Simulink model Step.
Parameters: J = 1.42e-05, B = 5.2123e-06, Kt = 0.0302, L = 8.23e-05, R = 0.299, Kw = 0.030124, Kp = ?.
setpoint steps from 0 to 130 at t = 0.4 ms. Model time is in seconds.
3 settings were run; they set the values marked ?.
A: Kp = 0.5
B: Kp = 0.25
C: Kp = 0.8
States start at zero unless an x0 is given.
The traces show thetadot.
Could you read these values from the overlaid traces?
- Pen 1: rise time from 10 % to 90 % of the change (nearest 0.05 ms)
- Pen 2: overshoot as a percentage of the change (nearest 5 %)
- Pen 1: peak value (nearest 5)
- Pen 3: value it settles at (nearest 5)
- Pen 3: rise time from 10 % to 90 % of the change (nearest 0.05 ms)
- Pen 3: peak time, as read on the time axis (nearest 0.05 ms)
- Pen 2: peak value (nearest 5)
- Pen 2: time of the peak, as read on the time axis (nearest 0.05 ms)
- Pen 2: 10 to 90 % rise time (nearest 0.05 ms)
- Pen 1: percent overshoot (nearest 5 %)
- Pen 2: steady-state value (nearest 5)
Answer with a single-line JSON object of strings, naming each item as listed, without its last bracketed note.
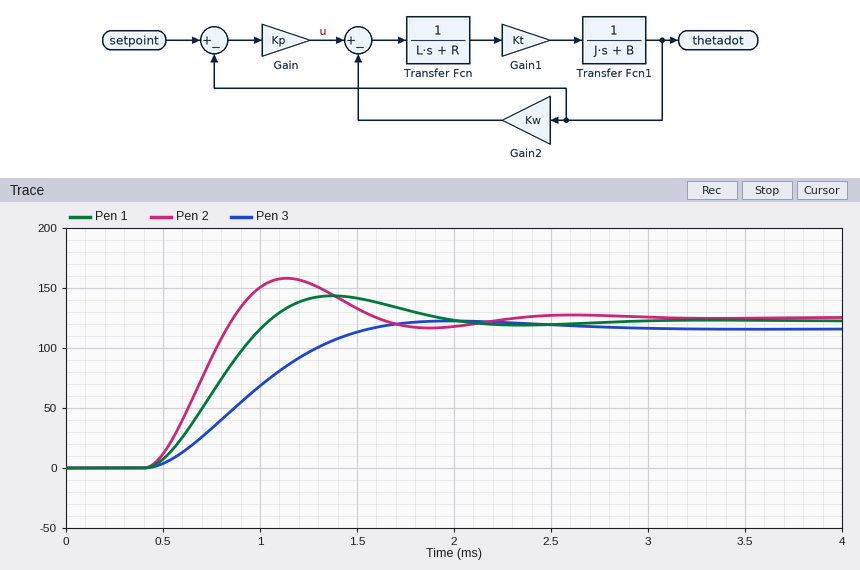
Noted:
{"Pen 1: rise time from 10 % to 90 % of the change": "0.45 ms", "Pen 2: overshoot as a percentage of the change": "25 %", "Pen 1: peak value": "145", "Pen 3: value it settles at": "115", "Pen 3: rise time from 10 % to 90 % of the change": "0.75 ms", "Pen 3: peak time, as read on the time axis": "2.00 ms", "Pen 2: peak value": "160", "Pen 2: time of the peak, as read on the time axis": "1.15 ms", "Pen 2: 10 to 90 % rise time": "0.30 ms", "Pen 1: percent overshoot": "15 %", "Pen 2: steady-state value": "125"}
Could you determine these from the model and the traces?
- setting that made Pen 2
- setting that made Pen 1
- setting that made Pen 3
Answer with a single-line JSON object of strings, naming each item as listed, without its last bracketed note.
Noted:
{"setting that made Pen 2": "C", "setting that made Pen 1": "A", "setting that made Pen 3": "B"}
